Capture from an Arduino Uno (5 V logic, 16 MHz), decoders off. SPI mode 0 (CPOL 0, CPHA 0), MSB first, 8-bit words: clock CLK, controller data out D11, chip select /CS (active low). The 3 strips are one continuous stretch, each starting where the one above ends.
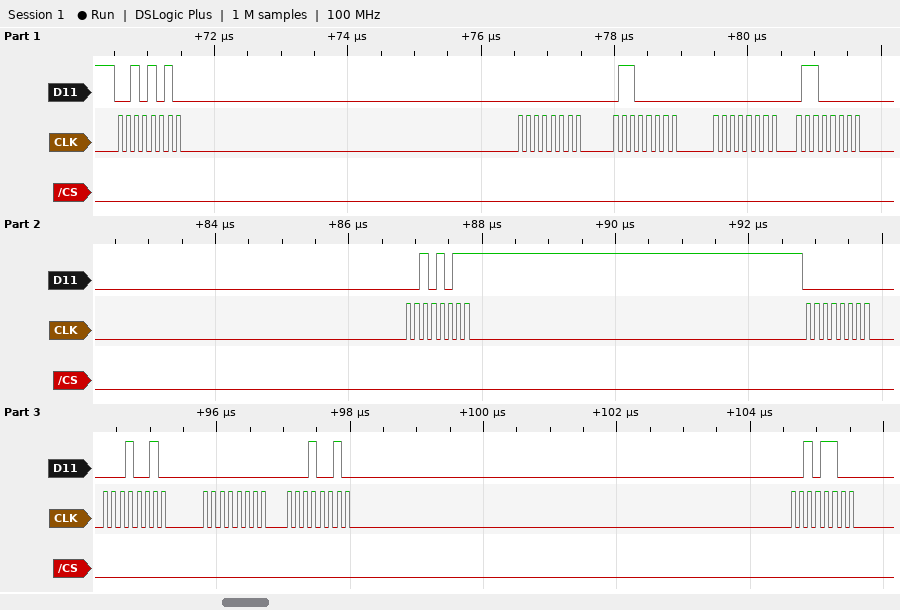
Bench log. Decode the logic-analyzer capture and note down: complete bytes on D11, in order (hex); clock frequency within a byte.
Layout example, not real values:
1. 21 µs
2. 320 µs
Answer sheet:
1. 2A 00 60 00 60 2B 00 12 00 12 2C
2. 8 MHz
